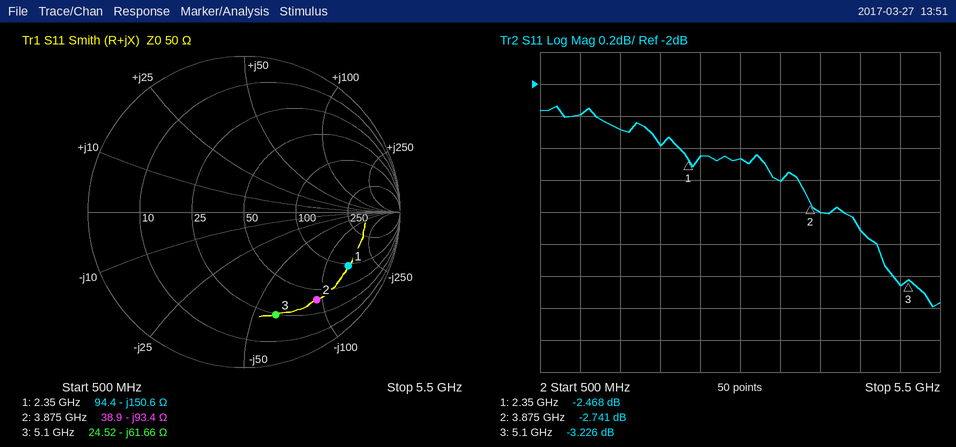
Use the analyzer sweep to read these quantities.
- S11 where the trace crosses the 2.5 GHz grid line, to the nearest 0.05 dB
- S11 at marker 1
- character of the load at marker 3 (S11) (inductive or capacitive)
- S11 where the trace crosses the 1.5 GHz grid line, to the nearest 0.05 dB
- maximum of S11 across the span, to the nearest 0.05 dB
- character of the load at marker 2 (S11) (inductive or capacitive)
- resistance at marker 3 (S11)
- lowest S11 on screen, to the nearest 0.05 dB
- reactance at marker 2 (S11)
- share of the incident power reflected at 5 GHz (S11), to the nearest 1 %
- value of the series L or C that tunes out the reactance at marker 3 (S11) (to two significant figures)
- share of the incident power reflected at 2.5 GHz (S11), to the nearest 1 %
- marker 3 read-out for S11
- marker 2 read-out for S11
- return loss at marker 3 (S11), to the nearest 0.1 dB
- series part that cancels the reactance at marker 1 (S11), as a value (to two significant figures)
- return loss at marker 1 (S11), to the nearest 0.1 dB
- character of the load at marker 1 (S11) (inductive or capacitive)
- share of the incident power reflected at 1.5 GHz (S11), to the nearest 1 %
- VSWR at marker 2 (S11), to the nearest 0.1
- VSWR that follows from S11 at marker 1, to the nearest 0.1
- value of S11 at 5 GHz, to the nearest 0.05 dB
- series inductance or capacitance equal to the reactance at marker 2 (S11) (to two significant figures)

-2.45 dB
-2.468 dB
capacitive
-2.30 dB
-2.15 dB
capacitive
24.52 Ω
-3.40 dB
-93.4 Ω
47 %
1.9 nH
57 %
-3.226 dB
-2.741 dB
3.2 dB
10 nH
2.5 dB
capacitive
59 %
6.4
7.1
-3.25 dB
440 fF
